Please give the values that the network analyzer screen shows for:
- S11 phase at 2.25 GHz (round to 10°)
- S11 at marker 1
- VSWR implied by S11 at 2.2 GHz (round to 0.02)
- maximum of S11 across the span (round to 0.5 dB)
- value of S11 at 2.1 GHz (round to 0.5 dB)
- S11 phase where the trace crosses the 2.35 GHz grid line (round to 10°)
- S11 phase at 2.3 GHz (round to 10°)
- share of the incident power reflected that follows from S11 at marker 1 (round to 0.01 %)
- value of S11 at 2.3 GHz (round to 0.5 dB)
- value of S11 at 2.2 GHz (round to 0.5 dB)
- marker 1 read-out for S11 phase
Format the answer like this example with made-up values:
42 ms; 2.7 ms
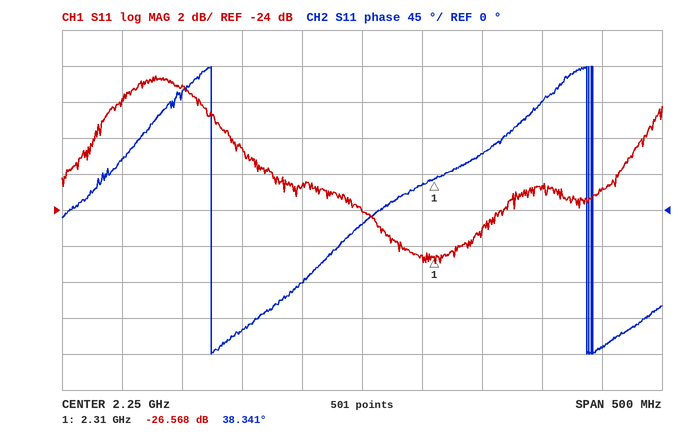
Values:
-20°; -26.568 dB; 1.16; -16.5 dB; -17.0 dB; 70°; 30°; 0.22 %; -26.5 dB; -22.5 dB; 38.341°
